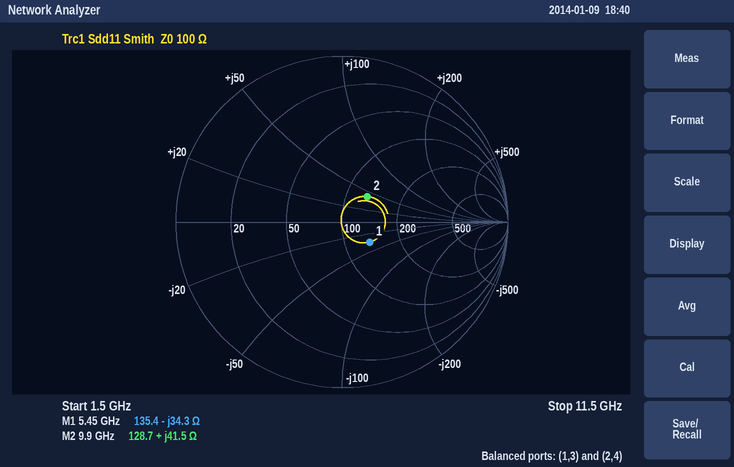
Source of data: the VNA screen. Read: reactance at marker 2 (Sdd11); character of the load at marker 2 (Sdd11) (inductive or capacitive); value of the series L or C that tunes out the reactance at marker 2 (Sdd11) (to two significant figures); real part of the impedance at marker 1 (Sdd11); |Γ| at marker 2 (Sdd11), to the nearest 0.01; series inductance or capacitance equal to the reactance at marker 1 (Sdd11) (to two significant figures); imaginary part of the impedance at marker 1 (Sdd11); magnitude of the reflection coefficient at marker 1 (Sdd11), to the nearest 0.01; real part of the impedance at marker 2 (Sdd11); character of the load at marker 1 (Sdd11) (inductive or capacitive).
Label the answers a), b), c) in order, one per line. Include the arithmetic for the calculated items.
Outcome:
a) +41.5 Ω
b) inductive
c) C = 1/(2π × 9.9 GHz × 41.5 Ω) ≈ 387 fF, so 390 fF to two significant figures
d) 135.4 Ω
e) 0.22
f) C = 1/(2π × 5.45 GHz × 34.3 Ω) ≈ 851 fF, so 850 fF to two significant figures
g) -34.3 Ω
h) 0.21
i) 128.7 Ω
j) capacitive
